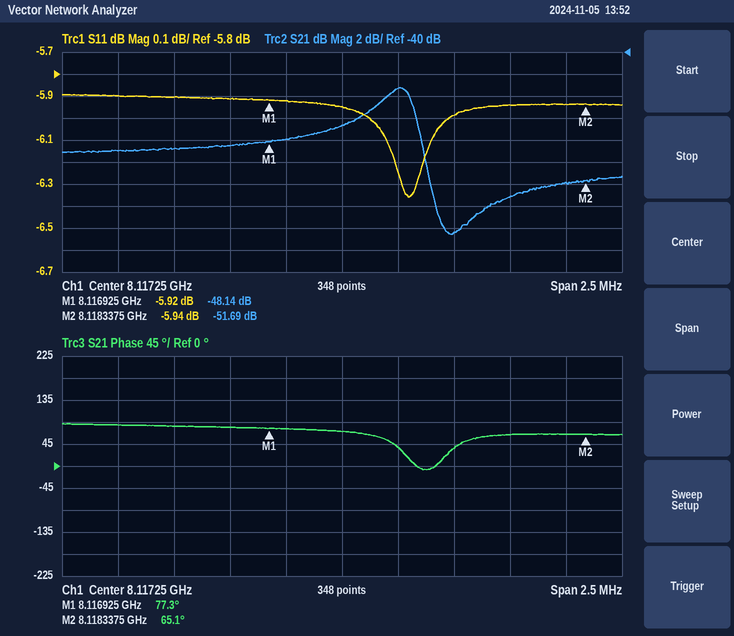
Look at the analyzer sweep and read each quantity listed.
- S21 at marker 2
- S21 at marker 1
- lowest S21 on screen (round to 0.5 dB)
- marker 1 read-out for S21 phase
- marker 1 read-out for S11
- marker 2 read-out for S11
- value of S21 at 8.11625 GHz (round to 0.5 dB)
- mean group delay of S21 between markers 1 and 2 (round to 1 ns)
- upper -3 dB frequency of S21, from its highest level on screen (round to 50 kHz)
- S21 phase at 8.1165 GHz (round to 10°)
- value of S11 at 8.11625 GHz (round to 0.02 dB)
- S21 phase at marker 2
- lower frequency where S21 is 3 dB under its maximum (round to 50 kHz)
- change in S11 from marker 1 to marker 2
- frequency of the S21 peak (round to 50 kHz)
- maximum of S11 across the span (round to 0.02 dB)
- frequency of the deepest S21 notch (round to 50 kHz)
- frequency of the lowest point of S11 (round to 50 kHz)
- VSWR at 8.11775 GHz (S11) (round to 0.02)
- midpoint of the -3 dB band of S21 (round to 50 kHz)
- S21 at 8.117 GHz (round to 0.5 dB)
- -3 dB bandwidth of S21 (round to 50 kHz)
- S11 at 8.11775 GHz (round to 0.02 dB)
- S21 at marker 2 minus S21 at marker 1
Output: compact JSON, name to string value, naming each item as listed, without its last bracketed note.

{"S21 at marker 2": "-51.69 dB", "S21 at marker 1": "-48.14 dB", "lowest S21 on screen": "-56.5 dB", "marker 1 read-out for S21 phase": "77.3°", "marker 1 read-out for S11": "-5.92 dB", "marker 2 read-out for S11": "-5.94 dB", "value of S21 at 8.11625 GHz": "-49.0 dB", "mean group delay of S21 between markers 1 and 2": "24 ns", "upper -3 dB frequency of S21, from its highest level on screen": "8.11760 GHz", "S21 phase at 8.1165 GHz": "80°", "value of S11 at 8.11625 GHz": "-5.90 dB", "S21 phase at marker 2": "65.1°", "lower frequency where S21 is 3 dB under its maximum": "8.11730 GHz", "change in S11 from marker 1 to marker 2": "-0.02 dB", "frequency of the S21 peak": "8.11750 GHz", "maximum of S11 across the span": "-5.90 dB", "frequency of the deepest S21 notch": "8.11775 GHz", "frequency of the lowest point of S11": "8.11755 GHz", "VSWR at 8.11775 GHz (S11)": "3.02", "midpoint of the -3 dB band of S21": "8.11745 GHz", "S21 at 8.117 GHz": "-48.0 dB", "-3 dB bandwidth of S21": "300 kHz", "S11 at 8.11775 GHz": "-5.98 dB", "S21 at marker 2 minus S21 at marker 1": "-3.55 dB"}
